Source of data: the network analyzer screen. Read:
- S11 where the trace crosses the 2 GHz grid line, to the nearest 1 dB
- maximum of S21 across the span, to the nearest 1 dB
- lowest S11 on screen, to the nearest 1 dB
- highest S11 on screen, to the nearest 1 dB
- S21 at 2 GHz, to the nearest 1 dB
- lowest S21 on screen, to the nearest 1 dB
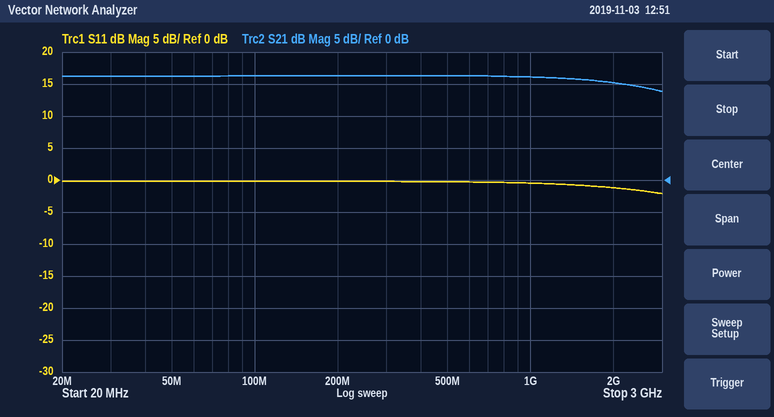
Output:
-1 dB
16 dB
-2 dB
0 dB
15 dB
14 dB
